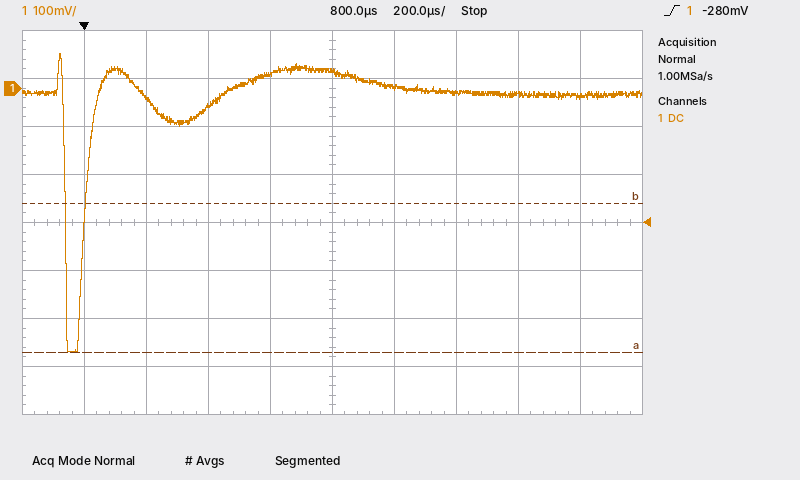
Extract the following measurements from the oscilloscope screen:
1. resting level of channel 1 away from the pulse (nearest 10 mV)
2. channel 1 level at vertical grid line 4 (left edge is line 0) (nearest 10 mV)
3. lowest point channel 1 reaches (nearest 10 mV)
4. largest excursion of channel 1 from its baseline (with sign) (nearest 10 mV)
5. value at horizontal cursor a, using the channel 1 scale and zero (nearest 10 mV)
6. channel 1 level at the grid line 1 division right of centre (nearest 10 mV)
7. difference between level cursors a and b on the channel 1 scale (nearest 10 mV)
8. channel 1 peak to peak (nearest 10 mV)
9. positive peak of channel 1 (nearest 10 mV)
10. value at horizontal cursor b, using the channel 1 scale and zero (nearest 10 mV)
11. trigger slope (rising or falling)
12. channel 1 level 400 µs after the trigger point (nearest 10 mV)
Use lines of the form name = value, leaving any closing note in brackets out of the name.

resting level of channel 1 away from the pulse = -10 mV
channel 1 level at vertical grid line 4 (left edge is line 0) = 30 mV
lowest point channel 1 reaches = -550 mV
largest excursion of channel 1 from its baseline (with sign) = -540 mV
value at horizontal cursor a, using the channel 1 scale and zero = -550 mV
channel 1 level at the grid line 1 division right of centre = 0 mV
difference between level cursors a and b on the channel 1 scale = 310 mV
channel 1 peak to peak = 620 mV
positive peak of channel 1 = 70 mV
value at horizontal cursor b, using the channel 1 scale and zero = -240 mV
trigger slope = rising
channel 1 level 400 µs after the trigger point = -40 mV
